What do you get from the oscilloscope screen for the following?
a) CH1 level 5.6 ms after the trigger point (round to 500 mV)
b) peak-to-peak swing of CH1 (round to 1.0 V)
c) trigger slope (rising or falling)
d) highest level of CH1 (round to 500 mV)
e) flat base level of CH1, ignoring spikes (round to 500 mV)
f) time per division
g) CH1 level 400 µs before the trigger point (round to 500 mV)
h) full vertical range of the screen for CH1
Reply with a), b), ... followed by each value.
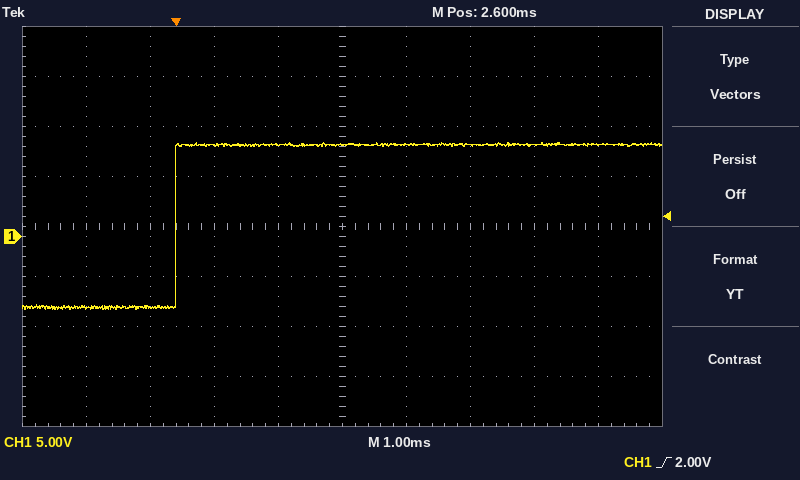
a) 9.0 V
b) 17.0 V
c) rising
d) 9.5 V
e) -7.0 V
f) 1 ms
g) -7.0 V
h) 40 V
